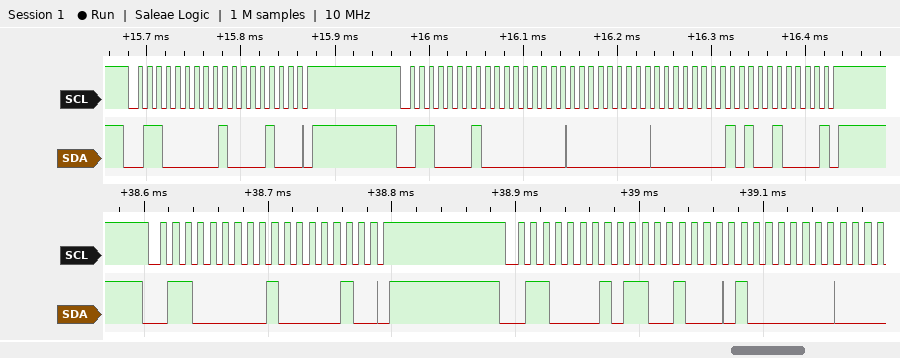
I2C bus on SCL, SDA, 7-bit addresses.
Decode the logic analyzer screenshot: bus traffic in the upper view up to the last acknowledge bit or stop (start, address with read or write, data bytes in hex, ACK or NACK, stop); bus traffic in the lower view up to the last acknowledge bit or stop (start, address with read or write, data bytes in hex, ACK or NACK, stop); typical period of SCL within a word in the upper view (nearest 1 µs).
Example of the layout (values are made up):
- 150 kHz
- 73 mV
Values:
- start, address 30 write ACK, 84 ACK, stop, start, address 30 read ACK, 00 ACK, 00 ACK, 01 ACK, 90 NACK, stop
- start, address 30 write ACK, 82 ACK, stop, start, address 30 read ACK, C8 ACK, 80 ACK
- 10 µs
